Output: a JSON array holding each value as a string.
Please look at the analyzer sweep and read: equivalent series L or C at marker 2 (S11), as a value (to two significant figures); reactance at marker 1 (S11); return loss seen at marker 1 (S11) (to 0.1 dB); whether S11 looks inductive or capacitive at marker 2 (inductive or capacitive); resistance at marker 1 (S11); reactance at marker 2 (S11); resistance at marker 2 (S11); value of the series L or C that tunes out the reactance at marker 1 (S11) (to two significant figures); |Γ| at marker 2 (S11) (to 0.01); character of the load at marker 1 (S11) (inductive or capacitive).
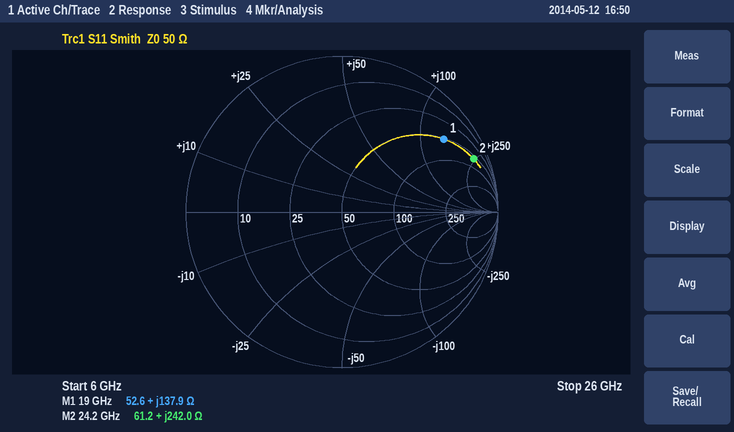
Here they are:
["1.6 nH", "+137.9 Ω", "1.9 dB", "inductive", "52.6 Ω", "+242.0 Ω", "61.2 Ω", "61 fF", "0.91", "inductive"]
